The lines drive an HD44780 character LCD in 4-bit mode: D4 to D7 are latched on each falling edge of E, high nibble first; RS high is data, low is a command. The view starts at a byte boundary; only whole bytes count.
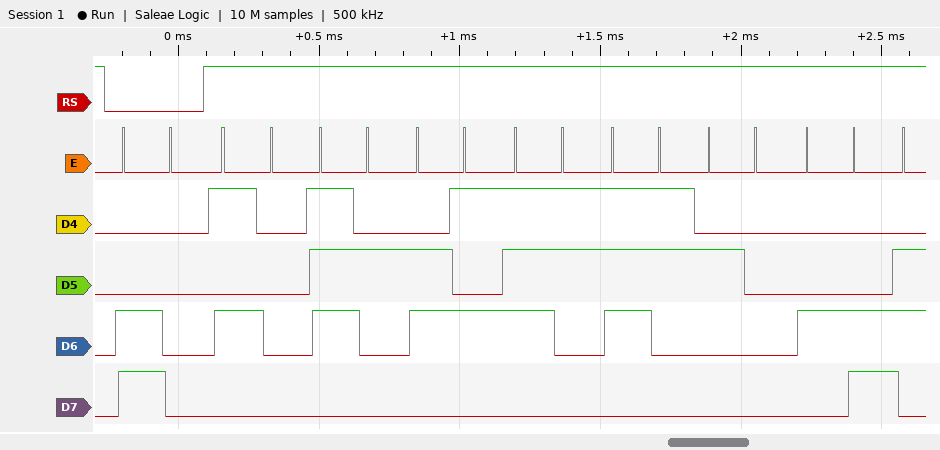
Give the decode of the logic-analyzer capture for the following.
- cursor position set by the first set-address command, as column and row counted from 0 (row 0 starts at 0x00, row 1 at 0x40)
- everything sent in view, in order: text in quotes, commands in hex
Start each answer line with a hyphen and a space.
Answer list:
- column 0, row 1
- 0xC0 "Press L"
